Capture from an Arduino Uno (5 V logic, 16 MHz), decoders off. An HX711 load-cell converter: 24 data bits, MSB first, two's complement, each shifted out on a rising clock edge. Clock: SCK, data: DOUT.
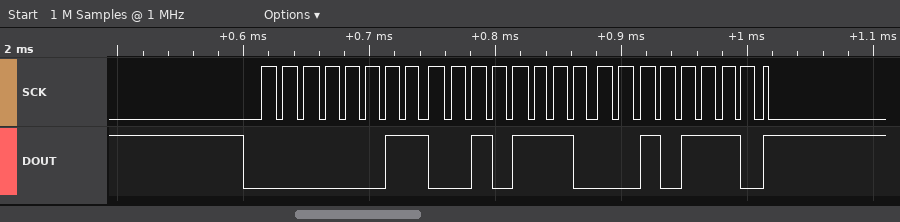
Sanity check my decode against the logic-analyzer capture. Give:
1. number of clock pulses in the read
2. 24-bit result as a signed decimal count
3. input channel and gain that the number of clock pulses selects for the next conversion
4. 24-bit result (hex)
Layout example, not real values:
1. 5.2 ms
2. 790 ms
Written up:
1. 25
2. 208430
3. channel A, gain 128
4. 0x032E2E
